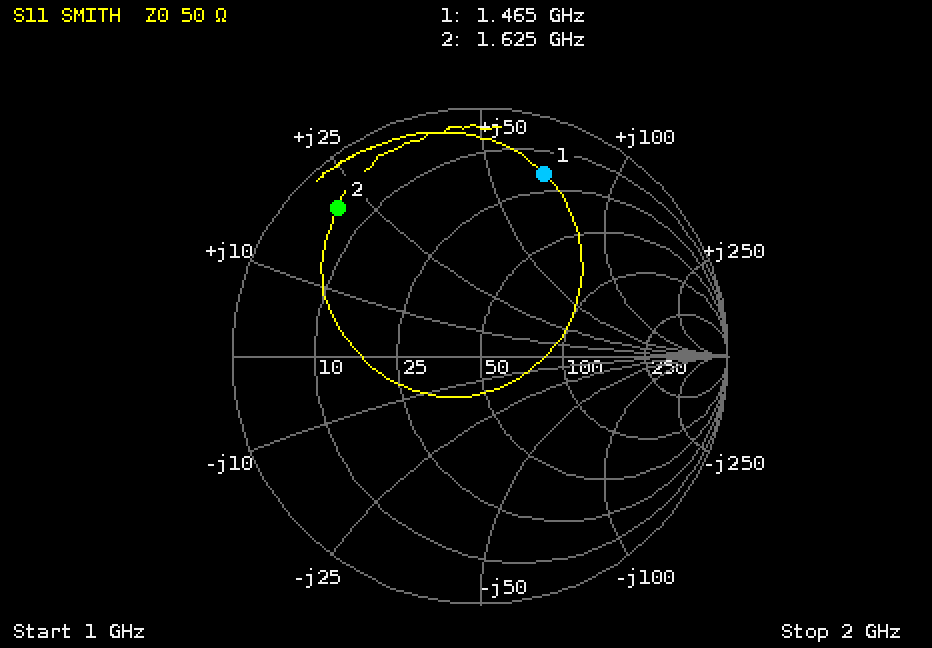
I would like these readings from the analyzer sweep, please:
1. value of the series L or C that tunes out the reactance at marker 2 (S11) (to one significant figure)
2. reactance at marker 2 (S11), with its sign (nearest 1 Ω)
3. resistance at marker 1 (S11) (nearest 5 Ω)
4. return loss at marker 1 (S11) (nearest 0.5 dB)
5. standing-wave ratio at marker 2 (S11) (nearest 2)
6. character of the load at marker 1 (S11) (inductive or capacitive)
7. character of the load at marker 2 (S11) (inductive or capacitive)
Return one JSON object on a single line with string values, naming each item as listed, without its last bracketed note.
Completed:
{"value of the series L or C that tunes out the reactance at marker 2 (S11)": "5 pF", "reactance at marker 2 (S11), with its sign": "+21 Ω", "resistance at marker 1 (S11)": "20 Ω", "return loss at marker 1 (S11)": "2.0 dB", "standing-wave ratio at marker 2 (S11)": "10", "character of the load at marker 1 (S11)": "inductive", "character of the load at marker 2 (S11)": "inductive"}
